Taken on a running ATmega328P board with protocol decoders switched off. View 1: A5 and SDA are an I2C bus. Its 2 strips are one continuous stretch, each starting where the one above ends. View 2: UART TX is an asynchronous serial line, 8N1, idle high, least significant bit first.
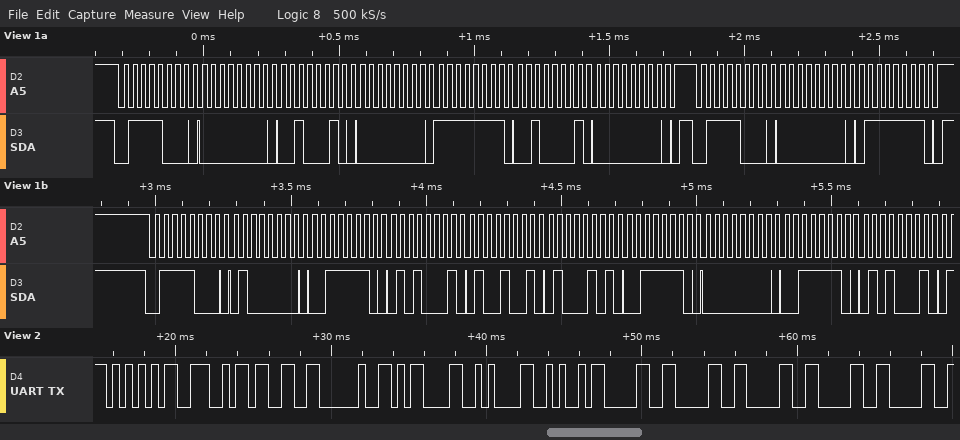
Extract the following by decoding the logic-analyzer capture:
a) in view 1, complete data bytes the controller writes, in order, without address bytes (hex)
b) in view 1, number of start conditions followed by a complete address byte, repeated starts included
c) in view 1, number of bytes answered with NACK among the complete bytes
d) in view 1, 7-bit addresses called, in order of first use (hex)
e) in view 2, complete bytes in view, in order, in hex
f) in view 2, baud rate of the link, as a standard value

00 22 00 FF 21 00 00 7F 40 3E 51 49 45 3E 00 3E 51
3
0
0x3C
55 4E 33 20 0D 0A 4A 30 30 30 30 30
2400 baud
